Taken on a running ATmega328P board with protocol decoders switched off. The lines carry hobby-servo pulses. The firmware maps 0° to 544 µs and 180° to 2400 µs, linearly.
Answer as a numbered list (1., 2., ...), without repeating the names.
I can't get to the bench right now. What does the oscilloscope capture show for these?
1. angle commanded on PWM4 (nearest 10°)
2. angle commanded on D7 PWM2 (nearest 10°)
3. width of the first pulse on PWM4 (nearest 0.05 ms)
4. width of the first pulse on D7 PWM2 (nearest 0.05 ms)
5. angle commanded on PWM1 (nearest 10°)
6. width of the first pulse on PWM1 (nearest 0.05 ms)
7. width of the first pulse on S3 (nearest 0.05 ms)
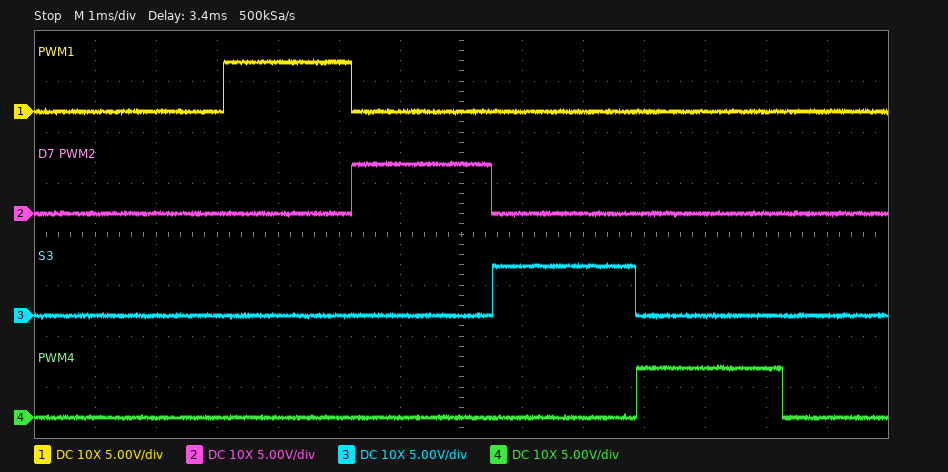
1. 180°
2. 170°
3. 2.40 ms
4. 2.30 ms
5. 150°
6. 2.10 ms
7. 2.35 ms
